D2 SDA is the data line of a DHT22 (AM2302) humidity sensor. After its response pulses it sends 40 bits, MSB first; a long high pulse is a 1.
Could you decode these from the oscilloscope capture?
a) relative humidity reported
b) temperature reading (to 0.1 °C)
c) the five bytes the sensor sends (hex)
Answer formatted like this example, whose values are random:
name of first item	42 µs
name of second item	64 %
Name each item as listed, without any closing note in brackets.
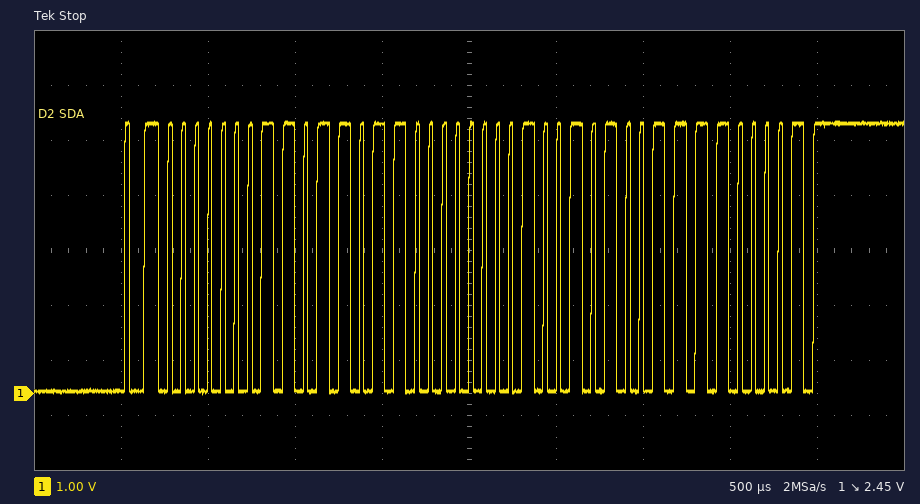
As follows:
relative humidity reported	43.8 %
temperature reading	29.7 °C
the five bytes the sensor sends	01 B6 01 29 E1
